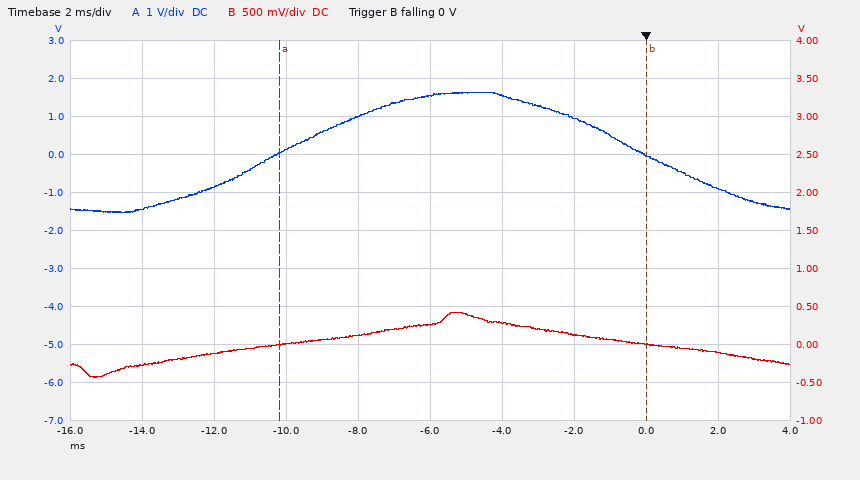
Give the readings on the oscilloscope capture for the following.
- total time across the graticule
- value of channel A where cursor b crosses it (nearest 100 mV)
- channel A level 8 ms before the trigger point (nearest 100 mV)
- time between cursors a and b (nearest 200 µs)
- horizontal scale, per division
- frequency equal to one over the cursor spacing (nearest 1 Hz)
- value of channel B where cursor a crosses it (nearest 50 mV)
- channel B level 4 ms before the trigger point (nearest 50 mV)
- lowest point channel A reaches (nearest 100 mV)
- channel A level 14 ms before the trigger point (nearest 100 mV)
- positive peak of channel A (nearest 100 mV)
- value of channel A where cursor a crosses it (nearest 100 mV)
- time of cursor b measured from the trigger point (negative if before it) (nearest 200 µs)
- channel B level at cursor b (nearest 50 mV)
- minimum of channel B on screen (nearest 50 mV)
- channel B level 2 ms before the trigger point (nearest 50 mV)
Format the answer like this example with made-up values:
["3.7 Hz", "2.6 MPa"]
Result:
["20 ms", "0.0 V", "1.0 V", "10.2 ms", "2 ms", "98 Hz", "0 mV", "300 mV", "-1.5 V", "-1.4 V", "1.6 V", "0.0 V", "0.0 ms", "0 mV", "-450 mV", "150 mV"]
